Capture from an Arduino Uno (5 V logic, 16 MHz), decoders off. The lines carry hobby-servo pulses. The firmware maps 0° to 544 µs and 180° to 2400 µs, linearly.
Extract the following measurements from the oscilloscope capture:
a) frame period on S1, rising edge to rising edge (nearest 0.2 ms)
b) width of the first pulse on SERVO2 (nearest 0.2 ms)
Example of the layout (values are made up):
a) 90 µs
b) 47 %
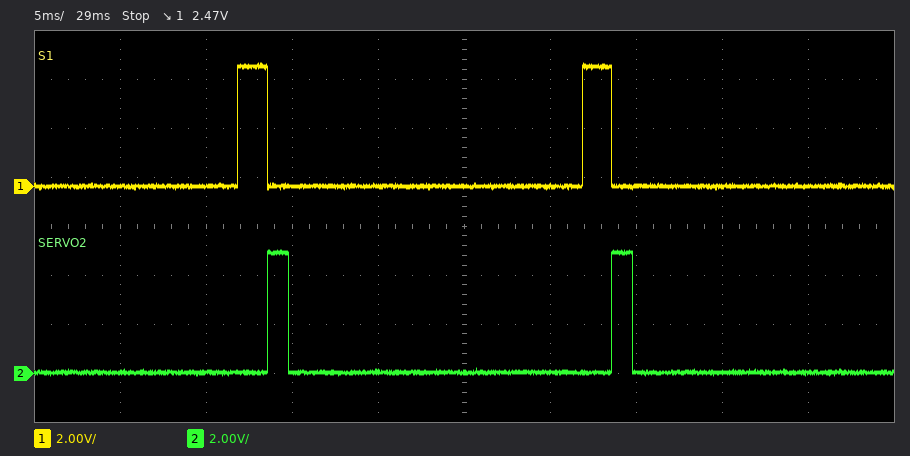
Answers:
a) 20.0 ms
b) 1.2 ms
